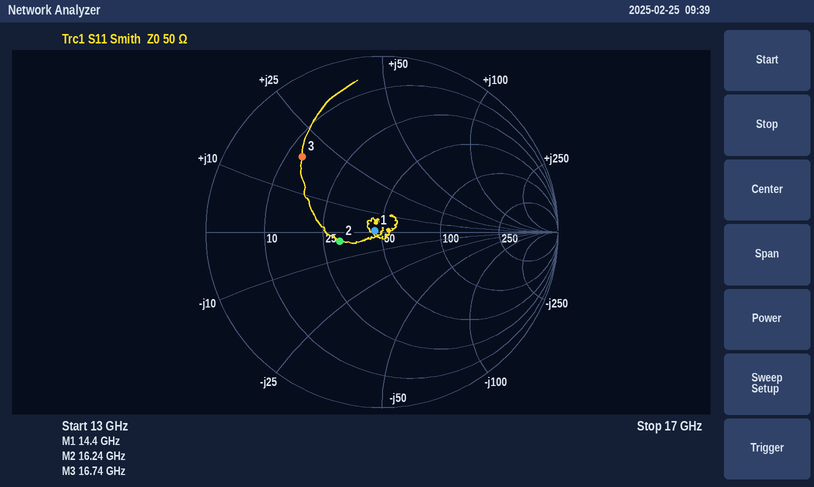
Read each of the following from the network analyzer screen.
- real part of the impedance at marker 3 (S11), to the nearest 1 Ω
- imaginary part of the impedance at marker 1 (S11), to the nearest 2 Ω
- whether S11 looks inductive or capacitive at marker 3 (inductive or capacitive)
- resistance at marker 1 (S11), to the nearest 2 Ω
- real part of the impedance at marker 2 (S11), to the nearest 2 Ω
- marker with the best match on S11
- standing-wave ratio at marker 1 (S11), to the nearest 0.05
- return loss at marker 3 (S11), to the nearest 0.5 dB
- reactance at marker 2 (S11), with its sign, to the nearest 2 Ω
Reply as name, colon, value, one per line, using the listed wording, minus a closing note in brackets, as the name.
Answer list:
real part of the impedance at marker 3 (S11), to the nearest 1 Ω: 13 Ω
imaginary part of the impedance at marker 1 (S11), to the nearest 2 Ω: 0 Ω
whether S11 looks inductive or capacitive at marker 3: inductive
resistance at marker 1 (S11), to the nearest 2 Ω: 46 Ω
real part of the impedance at marker 2 (S11), to the nearest 2 Ω: 30 Ω
marker with the best match on S11: marker 1
standing-wave ratio at marker 1 (S11), to the nearest 0.05: 1.10
return loss at marker 3 (S11), to the nearest 0.5 dB: 4.0 dB
reactance at marker 2 (S11), with its sign, to the nearest 2 Ω: -4 Ω
